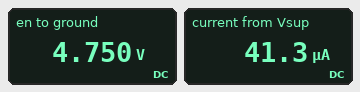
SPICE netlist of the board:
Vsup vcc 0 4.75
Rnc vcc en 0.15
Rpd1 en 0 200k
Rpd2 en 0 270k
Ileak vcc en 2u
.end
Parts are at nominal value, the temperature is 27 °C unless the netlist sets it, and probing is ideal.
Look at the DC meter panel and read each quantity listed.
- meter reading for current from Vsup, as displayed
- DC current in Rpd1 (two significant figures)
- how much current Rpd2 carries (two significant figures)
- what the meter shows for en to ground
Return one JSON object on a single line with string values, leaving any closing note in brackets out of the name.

{"meter reading for current from Vsup, as displayed": "41.3 µA", "DC current in Rpd1": "24 µA", "how much current Rpd2 carries": "18 µA", "what the meter shows for en to ground": "4.750 V"}
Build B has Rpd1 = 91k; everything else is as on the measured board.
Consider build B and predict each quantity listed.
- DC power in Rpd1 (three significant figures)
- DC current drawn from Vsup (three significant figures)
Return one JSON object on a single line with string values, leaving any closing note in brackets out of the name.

{"DC power in Rpd1": "248 µW", "DC current drawn from Vsup": "69.8 µA"}
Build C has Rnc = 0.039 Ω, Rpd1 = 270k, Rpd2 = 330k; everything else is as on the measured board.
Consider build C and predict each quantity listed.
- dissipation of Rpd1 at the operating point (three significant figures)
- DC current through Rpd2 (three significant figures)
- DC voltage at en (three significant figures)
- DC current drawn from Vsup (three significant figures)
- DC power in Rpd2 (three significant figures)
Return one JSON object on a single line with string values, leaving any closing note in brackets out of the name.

{"dissipation of Rpd1 at the operating point": "83.6 µW", "DC current through Rpd2": "14.4 µA", "DC voltage at en": "4.75 V", "DC current drawn from Vsup": "32.0 µA", "DC power in Rpd2": "68.4 µW"}
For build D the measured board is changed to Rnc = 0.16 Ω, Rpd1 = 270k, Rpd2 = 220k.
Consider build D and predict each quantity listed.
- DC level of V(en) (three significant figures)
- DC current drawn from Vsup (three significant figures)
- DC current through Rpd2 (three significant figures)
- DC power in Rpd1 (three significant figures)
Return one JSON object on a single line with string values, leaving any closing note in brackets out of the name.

{"DC level of V(en)": "4.75 V", "DC current drawn from Vsup": "39.2 µA", "DC current through Rpd2": "21.6 µA", "DC power in Rpd1": "83.6 µW"}
